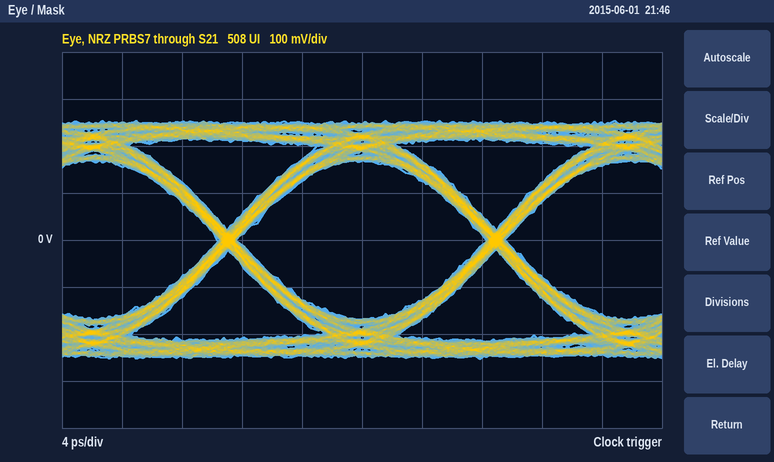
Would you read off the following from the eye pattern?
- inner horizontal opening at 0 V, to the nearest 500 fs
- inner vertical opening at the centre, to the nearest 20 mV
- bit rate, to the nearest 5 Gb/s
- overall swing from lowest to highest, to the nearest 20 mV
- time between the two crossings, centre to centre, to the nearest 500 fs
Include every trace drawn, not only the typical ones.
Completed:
16.5 ps
340 mV
55 Gb/s
500 mV
18.0 ps
